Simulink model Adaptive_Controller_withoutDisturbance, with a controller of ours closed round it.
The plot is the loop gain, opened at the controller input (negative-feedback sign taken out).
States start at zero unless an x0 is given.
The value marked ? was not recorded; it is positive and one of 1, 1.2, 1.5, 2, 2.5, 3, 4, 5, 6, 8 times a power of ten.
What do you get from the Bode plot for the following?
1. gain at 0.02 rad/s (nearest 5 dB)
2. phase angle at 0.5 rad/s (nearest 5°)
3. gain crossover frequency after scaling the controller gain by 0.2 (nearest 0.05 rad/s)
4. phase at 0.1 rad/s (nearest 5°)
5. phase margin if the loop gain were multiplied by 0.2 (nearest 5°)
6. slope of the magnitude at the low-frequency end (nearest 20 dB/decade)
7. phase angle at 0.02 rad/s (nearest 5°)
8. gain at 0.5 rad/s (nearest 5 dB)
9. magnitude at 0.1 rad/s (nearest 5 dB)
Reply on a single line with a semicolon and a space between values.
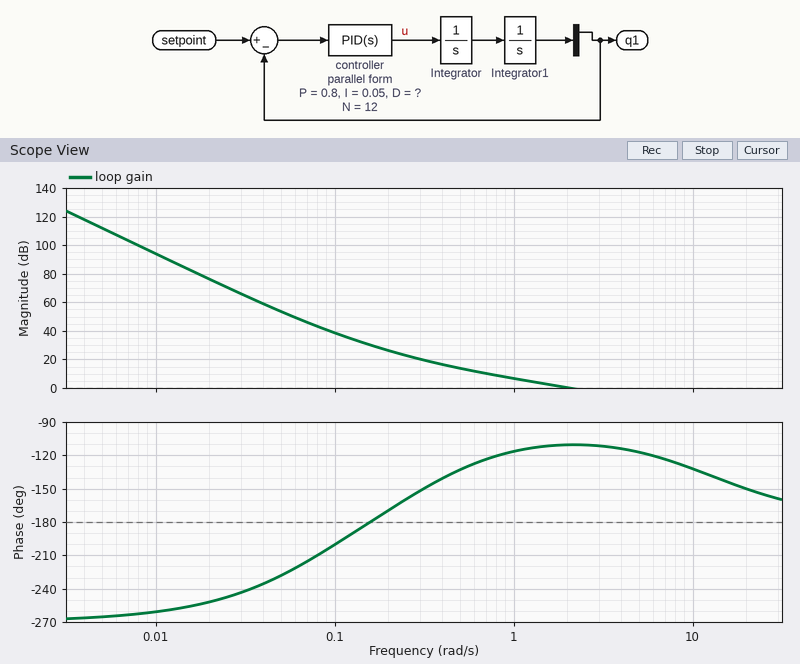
75 dB; -135°; 0.50 rad/s; -200°; 45°; -60 dB/decade; -250°; 15 dB; 40 dB
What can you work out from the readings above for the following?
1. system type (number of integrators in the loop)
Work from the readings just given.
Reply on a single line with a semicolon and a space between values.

3
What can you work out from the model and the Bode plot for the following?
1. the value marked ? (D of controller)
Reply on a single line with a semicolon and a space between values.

2
